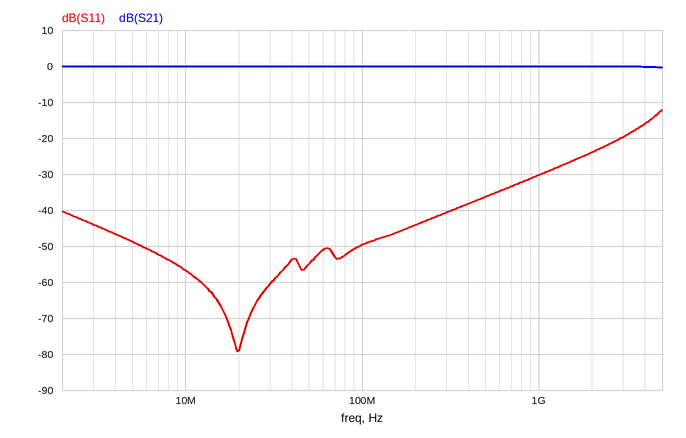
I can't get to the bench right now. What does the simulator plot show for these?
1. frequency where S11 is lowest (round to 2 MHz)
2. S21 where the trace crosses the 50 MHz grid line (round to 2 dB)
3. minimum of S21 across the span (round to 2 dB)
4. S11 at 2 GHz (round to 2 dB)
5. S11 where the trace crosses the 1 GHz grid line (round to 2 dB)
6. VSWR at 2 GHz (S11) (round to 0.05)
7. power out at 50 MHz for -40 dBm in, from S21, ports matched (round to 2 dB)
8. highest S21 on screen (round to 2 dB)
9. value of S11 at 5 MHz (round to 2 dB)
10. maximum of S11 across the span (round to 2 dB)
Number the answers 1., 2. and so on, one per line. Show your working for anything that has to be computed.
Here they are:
1. 20 MHz
2. 0 dB
3. 0 dB
4. -24 dB
5. -30 dB
6. |Γ| = 10^(-24/20) = 0.0631; VSWR = (1 + 0.0631)/(1 − 0.0631) ≈ 1.13, so 1.15 to the nearest 0.05
7. -40 dBm + (0 dB) = -40 dBm
8. 0 dB
9. -48 dB
10. -12 dB
